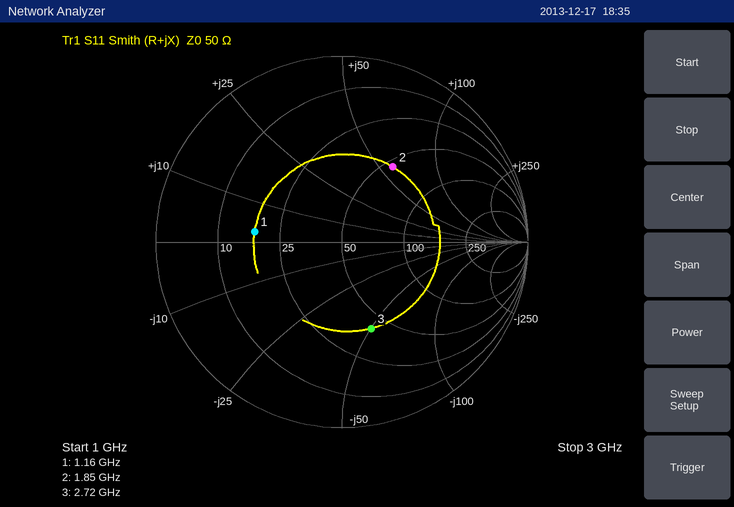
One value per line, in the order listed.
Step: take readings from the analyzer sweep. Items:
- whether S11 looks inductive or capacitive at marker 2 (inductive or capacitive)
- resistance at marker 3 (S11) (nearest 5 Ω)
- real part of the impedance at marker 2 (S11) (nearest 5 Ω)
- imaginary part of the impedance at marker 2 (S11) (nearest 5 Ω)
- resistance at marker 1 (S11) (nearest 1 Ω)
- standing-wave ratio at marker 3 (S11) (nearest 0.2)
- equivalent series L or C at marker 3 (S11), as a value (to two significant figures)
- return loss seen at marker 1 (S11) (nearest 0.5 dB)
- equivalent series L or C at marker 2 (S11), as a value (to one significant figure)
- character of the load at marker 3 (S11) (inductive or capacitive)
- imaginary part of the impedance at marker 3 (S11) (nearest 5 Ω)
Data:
inductive
40 Ω
55 Ω
+60 Ω
18 Ω
3.0
1.2 pF
6.5 dB
5 nH
capacitive
-50 Ω
